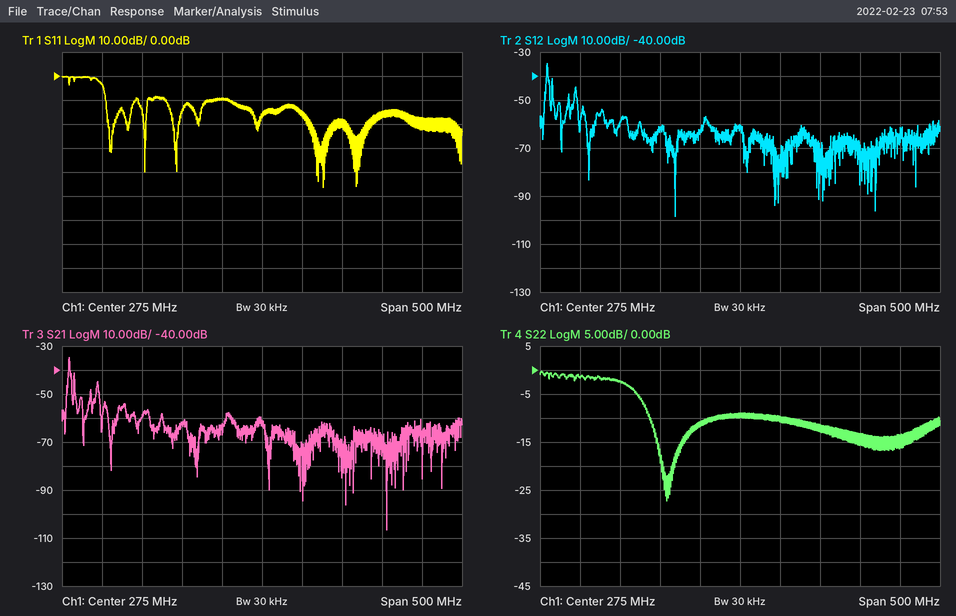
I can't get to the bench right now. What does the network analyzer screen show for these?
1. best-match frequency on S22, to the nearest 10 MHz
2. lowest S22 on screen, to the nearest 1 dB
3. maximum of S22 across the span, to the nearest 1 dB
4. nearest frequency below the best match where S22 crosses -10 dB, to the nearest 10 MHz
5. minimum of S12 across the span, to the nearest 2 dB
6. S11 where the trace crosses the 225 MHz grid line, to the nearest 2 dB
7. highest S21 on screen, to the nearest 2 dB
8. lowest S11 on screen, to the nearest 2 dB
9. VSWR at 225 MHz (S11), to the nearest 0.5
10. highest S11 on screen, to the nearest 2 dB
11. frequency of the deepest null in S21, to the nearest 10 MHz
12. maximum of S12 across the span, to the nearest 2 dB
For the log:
180 MHz
-27 dB
0 dB
160 MHz
-98 dB
-10 dB
-34 dB
-46 dB
2.0
0 dB
430 MHz
-34 dB
